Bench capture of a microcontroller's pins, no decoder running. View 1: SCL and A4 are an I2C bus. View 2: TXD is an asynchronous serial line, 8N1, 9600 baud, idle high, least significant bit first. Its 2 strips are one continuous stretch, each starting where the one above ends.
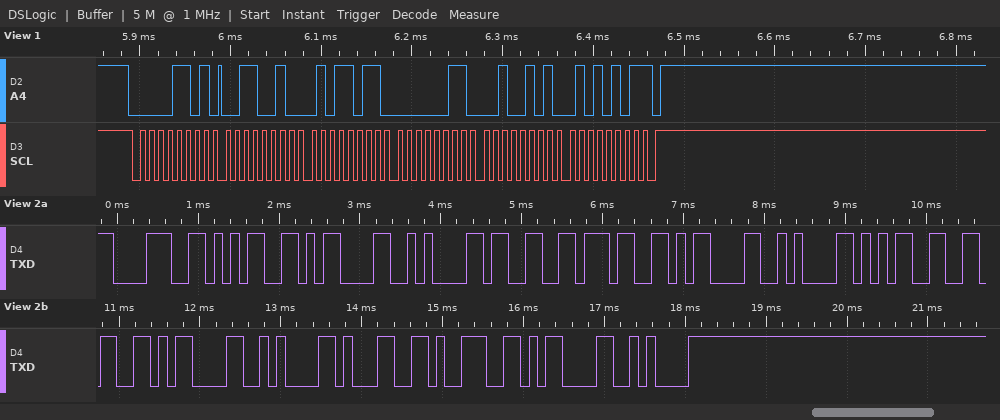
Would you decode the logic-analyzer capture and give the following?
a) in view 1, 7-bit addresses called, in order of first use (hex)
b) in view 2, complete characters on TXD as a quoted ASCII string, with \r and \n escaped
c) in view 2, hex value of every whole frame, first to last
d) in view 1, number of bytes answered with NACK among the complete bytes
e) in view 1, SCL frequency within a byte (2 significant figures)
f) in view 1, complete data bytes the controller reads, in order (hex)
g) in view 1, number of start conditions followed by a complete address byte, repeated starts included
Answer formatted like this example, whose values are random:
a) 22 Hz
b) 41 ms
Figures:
a) 0x06
b) "85\r\n37\r\n56\r\n19\r\n"
c) 0x38 0x35 0x0D 0x0A 0x33 0x37 0x0D 0x0A 0x35 0x36 0x0D 0x0A 0x31 0x39 0x0D 0x0A
d) 1
e) 100 kHz
f) 32 5B 03 25 55
g) 1
